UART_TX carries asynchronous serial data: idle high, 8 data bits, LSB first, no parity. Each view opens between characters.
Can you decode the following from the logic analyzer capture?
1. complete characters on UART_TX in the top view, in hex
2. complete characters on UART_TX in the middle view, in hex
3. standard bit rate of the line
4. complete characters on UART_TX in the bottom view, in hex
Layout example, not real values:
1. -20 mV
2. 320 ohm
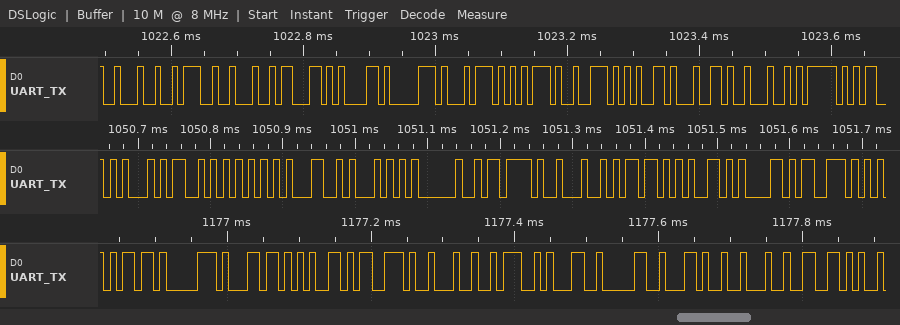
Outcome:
1. 22, 3A, 22, 63, 61, 70, 74, 75, 72, 65, 64, 22, 7D
2. 45, 53, 55, 4C, 54, 20, 7B, 22, 6D, 65, 61, 73
3. 115200 baud
4. 6D, 70, 6C, 65, 73, 22, 3A, 31, 30, 2C, 22, 66
